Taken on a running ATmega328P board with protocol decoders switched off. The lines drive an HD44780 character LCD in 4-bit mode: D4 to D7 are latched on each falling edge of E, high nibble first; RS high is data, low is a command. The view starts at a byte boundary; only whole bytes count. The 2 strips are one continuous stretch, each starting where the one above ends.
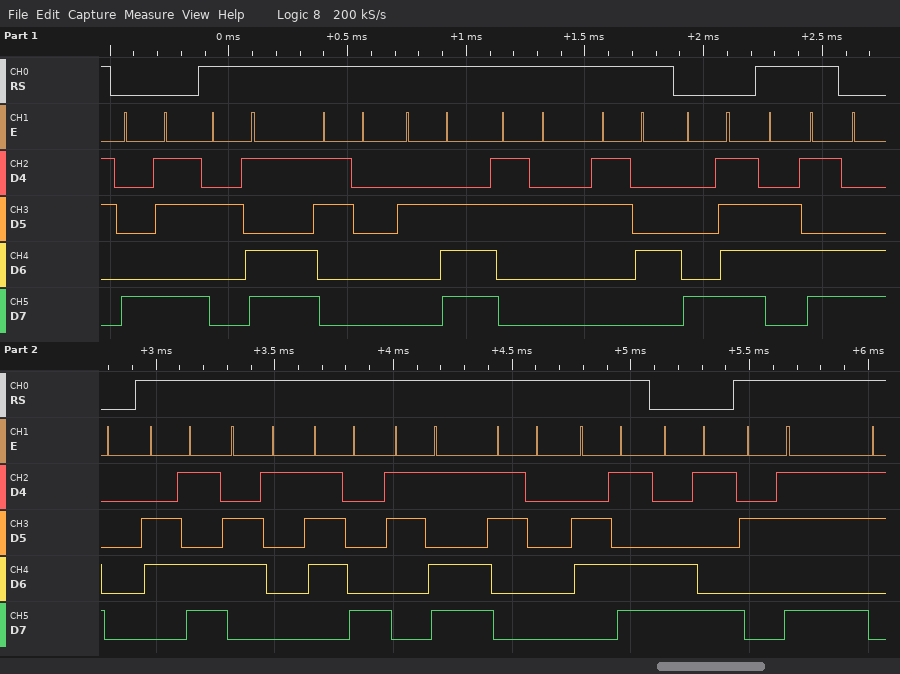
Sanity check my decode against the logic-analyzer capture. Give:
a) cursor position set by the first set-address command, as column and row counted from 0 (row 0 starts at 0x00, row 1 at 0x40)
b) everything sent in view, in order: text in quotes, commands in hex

column 11, row 0
0x8B "-0.24" 0x8F "m" 0xC0 "max=0m" 0xC9 "+"
